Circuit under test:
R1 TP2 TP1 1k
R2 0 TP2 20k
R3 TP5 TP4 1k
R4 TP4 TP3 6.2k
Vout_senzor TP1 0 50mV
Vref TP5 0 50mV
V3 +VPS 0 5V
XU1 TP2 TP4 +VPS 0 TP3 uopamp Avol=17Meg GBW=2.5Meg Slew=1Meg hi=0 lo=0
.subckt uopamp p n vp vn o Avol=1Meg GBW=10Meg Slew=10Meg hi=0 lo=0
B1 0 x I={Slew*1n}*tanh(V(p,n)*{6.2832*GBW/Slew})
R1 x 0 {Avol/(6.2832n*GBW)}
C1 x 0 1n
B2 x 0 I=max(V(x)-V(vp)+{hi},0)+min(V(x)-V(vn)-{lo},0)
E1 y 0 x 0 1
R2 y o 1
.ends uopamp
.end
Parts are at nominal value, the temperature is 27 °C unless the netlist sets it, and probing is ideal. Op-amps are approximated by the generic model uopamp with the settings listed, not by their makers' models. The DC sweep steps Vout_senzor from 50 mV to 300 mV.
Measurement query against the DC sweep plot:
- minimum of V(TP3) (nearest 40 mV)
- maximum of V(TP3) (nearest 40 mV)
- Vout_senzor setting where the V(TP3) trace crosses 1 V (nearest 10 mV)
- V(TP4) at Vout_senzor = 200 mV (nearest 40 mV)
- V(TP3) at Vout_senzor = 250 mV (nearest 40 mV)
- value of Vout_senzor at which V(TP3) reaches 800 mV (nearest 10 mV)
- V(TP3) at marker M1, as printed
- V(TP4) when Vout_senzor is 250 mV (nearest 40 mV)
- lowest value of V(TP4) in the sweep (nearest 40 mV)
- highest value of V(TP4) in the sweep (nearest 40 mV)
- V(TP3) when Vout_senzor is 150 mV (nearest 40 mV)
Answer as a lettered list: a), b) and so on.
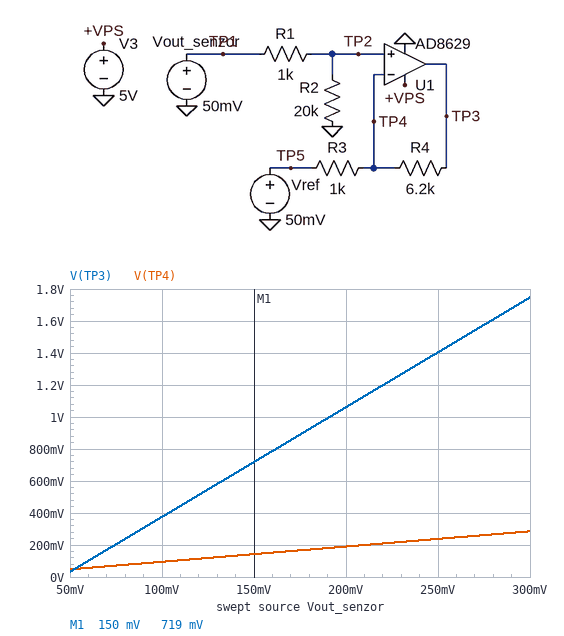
a) 40 mV
b) 1.76 V
c) 190 mV
d) 200 mV
e) 1.40 V
f) 160 mV
g) 719 mV
h) 240 mV
i) 40 mV
j) 280 mV
k) 720 mV
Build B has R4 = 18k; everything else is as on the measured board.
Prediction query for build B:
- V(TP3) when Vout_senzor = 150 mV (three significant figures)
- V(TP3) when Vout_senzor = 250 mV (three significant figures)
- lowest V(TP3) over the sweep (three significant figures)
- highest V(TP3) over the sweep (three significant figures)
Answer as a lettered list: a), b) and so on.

a) 1.81 V
b) 3.62 V
c) 4.76 mV
d) 4.53 V
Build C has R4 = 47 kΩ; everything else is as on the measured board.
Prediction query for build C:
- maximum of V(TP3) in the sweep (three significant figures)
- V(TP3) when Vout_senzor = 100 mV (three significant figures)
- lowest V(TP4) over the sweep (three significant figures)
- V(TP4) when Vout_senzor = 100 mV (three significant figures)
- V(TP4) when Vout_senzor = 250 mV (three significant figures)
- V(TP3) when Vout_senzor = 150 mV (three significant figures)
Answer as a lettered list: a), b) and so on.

a) 5.00 V
b) 2.22 V
c) 49.0 mV
d) 95.2 mV
e) 153 mV
f) 4.51 V
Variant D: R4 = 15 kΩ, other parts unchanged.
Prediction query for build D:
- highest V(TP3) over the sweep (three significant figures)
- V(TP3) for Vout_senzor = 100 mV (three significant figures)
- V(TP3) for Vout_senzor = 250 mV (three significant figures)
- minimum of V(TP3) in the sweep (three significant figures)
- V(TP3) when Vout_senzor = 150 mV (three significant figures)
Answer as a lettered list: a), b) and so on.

a) 3.82 V
b) 774 mV
c) 3.06 V
d) 11.9 mV
e) 1.54 V
